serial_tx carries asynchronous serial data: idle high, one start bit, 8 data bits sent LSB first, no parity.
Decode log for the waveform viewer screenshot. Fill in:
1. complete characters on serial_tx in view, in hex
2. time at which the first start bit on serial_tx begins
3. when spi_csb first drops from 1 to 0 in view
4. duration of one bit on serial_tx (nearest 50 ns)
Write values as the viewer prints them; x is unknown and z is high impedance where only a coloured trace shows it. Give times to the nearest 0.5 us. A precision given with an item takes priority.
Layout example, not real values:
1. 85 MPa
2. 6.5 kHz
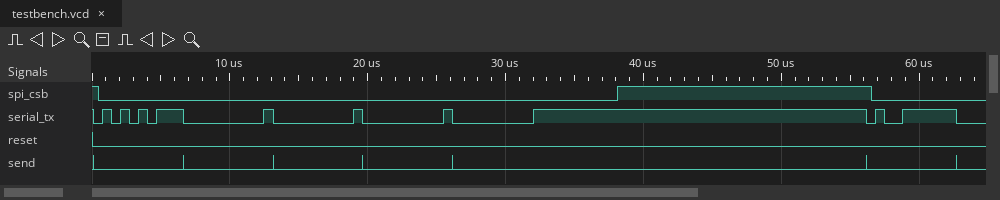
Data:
1. D5, 00, 00, 00, 00, F9
2. 0 us
3. 0.5 us
4. 650 ns
